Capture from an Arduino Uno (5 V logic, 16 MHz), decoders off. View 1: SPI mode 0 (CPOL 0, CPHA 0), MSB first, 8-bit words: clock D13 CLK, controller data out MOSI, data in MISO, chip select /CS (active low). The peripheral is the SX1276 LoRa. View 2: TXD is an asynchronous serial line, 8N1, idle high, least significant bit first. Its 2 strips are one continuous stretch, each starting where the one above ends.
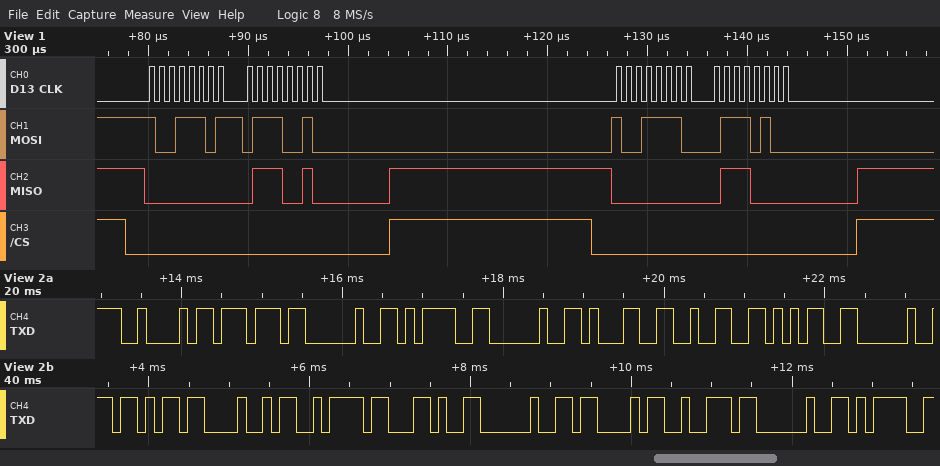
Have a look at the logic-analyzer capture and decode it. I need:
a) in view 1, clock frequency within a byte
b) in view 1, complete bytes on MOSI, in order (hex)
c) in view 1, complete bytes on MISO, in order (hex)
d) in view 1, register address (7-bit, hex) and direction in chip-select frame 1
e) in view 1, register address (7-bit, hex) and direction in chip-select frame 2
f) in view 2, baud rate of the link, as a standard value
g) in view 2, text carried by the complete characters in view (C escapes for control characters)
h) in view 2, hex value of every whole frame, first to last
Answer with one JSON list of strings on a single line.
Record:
["1 MHz", "9D 72 9E 74", "00 72 00 70", "0x1D write", "0x1E write", "9600 baud", "\"Bw = 125 kHz, Cr =\"", "0x42 0x77 0x20 0x3D 0x20 0x31 0x32 0x35 0x20 0x6B 0x48 0x7A 0x2C 0x20 0x43 0x72 0x20 0x3D"]
